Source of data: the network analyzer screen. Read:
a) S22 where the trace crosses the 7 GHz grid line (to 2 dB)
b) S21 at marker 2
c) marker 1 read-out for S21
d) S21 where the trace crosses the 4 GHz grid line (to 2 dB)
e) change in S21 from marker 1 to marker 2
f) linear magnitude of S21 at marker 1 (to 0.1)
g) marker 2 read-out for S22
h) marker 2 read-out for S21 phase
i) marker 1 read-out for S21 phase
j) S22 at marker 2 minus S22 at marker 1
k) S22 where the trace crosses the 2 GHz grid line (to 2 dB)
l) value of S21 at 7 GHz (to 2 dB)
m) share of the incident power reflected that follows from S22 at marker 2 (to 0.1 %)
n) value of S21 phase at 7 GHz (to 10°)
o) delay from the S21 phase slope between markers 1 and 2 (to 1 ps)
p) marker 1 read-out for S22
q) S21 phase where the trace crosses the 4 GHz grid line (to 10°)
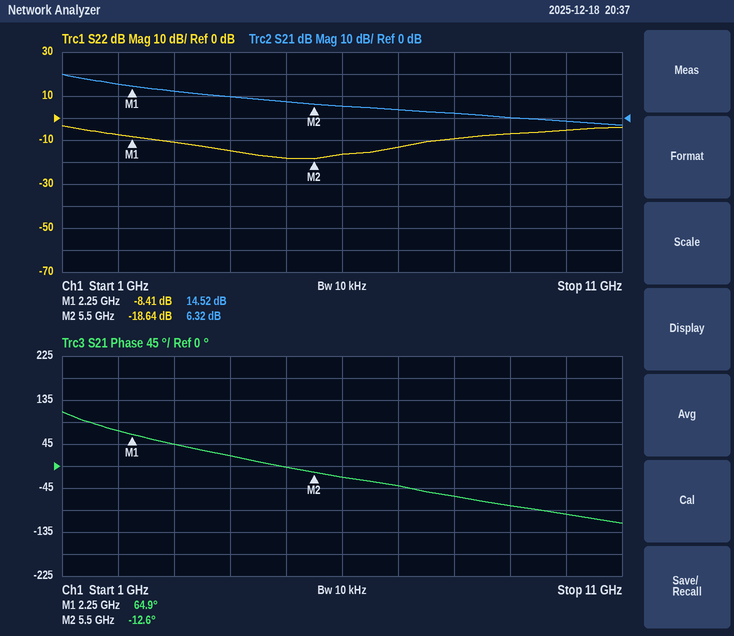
-14 dB
6.32 dB
14.52 dB
10 dB
-8.20 dB
5.3
-18.64 dB
-12.6°
64.9°
-10.23 dB
-8 dB
4 dB
1.4 %
-40°
66 ps
-8.41 dB
20°
